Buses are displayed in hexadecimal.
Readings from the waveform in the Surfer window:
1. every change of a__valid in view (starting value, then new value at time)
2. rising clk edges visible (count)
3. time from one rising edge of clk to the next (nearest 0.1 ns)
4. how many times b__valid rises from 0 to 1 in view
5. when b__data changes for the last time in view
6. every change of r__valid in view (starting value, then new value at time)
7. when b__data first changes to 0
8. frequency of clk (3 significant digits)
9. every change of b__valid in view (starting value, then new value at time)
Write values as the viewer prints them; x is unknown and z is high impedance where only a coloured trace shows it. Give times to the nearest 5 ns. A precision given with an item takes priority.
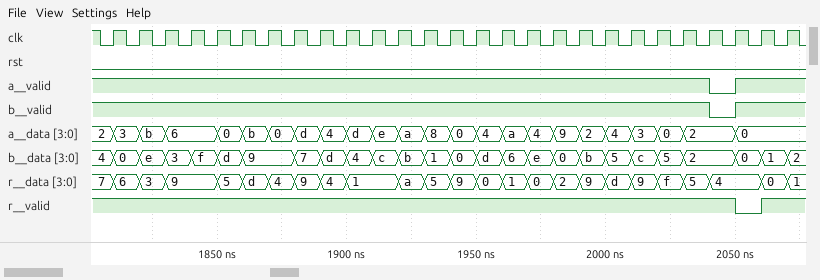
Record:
1, 0 at 2040 ns, 1 at 2050 ns
27
10 ns
1
2070 ns
1, 0 at 2050 ns, 1 at 2060 ns
1810 ns
100 MHz
1, 0 at 2040 ns, 1 at 2050 ns
